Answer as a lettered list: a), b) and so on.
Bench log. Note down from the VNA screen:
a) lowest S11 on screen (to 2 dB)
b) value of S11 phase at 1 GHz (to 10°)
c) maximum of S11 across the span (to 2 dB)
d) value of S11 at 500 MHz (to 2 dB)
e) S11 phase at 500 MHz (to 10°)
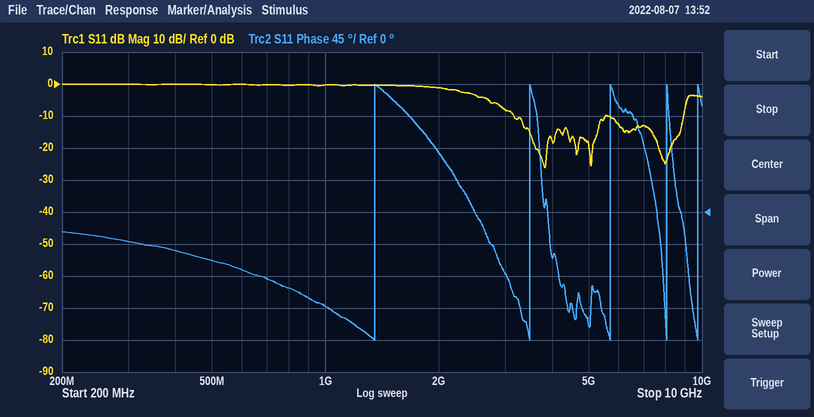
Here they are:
a) -26 dB
b) -130°
c) 0 dB
d) 0 dB
e) -70°
